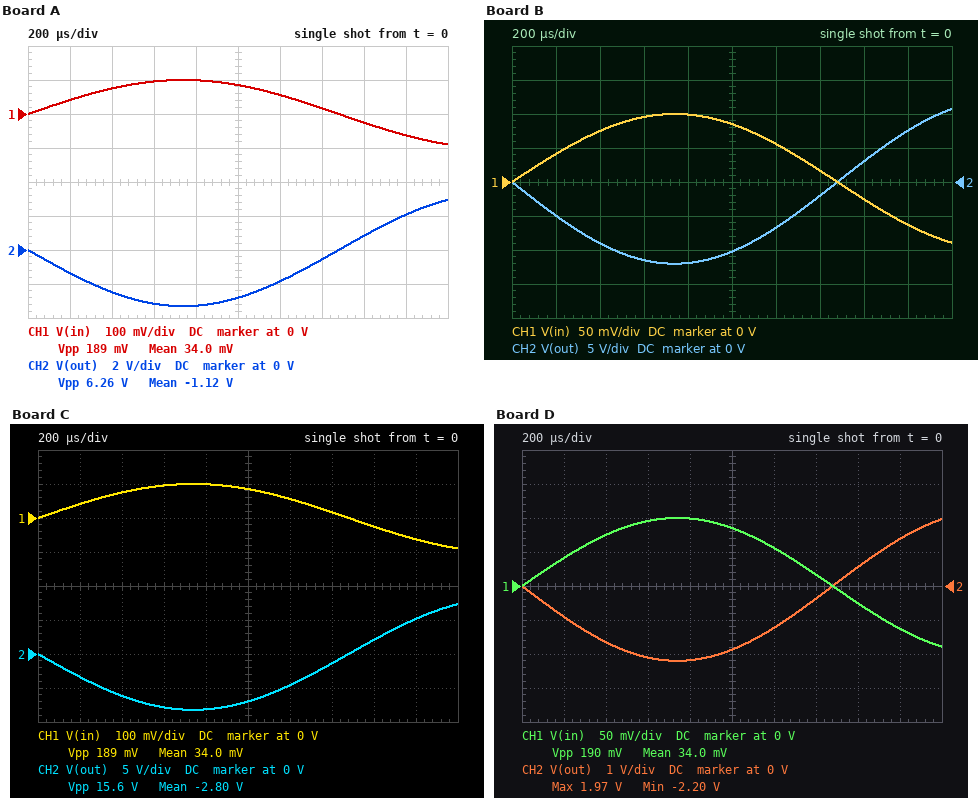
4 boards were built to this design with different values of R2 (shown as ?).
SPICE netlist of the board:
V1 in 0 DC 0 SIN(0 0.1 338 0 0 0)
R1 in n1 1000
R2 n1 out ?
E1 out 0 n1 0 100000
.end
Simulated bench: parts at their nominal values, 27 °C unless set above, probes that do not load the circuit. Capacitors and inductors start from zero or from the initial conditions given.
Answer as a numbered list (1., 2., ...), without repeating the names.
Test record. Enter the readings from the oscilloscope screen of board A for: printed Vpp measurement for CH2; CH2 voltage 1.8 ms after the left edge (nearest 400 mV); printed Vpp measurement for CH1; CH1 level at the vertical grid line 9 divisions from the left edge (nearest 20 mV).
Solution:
1. 6.26 V
2. 2.0 V
3. 189 mV
4. -60 mV
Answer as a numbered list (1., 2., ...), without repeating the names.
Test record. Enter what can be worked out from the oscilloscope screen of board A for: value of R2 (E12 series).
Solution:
1. 33 kΩ
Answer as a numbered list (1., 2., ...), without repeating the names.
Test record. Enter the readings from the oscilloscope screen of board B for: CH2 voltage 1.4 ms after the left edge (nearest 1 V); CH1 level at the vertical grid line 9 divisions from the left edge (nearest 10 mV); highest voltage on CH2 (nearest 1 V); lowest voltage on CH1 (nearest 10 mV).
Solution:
1. -2 V
2. -60 mV
3. 11 V
4. -90 mV
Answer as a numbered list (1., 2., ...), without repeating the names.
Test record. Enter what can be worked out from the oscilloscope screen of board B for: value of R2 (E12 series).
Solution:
1. 120 kΩ
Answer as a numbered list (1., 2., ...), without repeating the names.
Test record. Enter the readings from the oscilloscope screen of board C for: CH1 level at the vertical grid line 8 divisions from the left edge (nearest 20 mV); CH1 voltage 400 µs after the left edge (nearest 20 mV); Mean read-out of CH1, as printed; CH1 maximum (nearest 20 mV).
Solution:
1. -20 mV
2. 80 mV
3. 34.0 mV
4. 100 mV
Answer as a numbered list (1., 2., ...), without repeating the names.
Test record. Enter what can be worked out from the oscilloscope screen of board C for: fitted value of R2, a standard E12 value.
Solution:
1. 82 kΩ
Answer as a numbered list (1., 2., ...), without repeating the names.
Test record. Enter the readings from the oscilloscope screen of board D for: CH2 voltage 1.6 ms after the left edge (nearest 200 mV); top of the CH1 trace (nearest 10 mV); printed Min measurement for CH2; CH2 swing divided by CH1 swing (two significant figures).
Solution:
1. 600 mV
2. 100 mV
3. -2.20 V
4. 22
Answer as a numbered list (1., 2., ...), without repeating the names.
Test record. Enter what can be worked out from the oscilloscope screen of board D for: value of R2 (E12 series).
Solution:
1. 22 kΩ
